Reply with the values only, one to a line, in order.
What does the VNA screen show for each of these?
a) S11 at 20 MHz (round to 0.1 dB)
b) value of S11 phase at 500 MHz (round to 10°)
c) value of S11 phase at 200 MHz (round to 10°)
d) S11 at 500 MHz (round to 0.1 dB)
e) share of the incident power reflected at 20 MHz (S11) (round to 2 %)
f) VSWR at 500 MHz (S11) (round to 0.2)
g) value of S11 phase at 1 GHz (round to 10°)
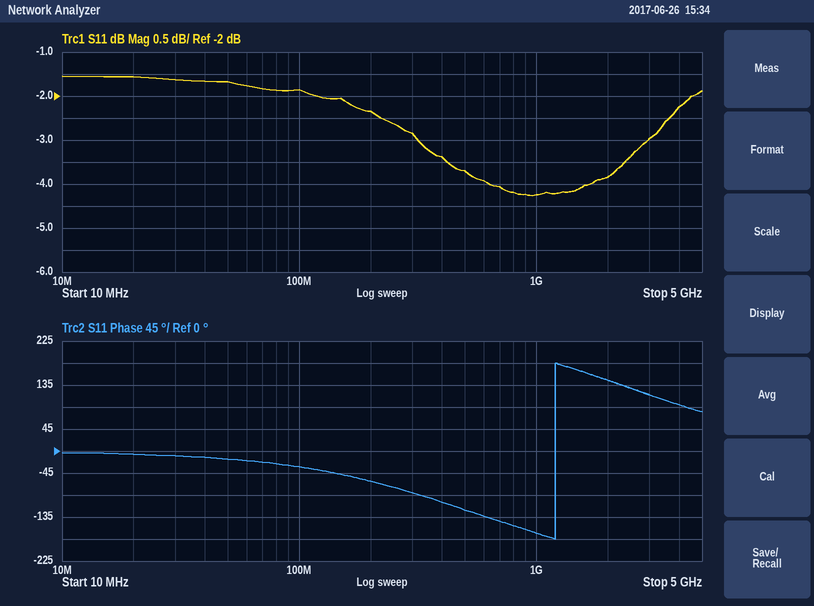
-1.6 dB
-120°
-60°
-3.7 dB
70 %
4.8
-170°
